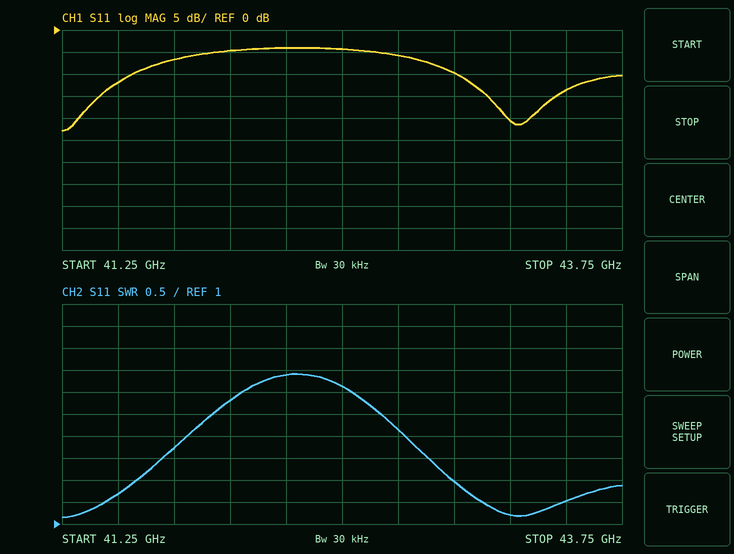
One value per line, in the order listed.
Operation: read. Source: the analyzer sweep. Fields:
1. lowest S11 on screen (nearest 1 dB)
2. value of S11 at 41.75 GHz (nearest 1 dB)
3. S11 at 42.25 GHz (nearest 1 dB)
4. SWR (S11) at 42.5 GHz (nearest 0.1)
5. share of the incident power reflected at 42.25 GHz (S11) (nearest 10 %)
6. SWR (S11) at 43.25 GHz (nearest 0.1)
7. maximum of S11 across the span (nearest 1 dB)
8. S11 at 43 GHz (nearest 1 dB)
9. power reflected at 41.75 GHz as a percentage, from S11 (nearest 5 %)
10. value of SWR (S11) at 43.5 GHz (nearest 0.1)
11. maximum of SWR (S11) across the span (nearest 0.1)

-23 dB
-7 dB
-4 dB
4.1
40 %
1.2
-4 dB
-10 dB
20 %
1.5
4.4
